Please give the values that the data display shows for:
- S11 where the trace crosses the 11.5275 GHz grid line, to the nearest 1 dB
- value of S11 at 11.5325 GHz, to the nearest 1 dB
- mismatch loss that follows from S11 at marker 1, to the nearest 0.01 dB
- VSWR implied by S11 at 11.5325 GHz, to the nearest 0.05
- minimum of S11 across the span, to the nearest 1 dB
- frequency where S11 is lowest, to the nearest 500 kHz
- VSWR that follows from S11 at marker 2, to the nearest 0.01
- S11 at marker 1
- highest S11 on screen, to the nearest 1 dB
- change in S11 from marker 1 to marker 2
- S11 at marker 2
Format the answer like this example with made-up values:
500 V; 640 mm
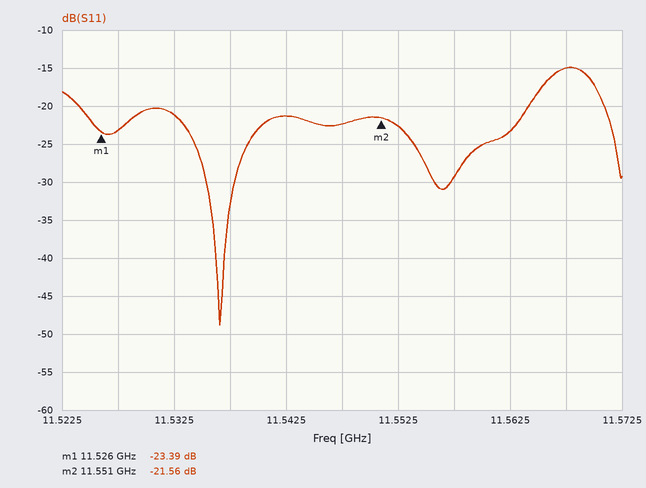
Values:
-23 dB; -21 dB; 0.02 dB; 1.20; -49 dB; 11.5365 GHz; 1.18; -23.39 dB; -15 dB; 1.83 dB; -21.56 dB
